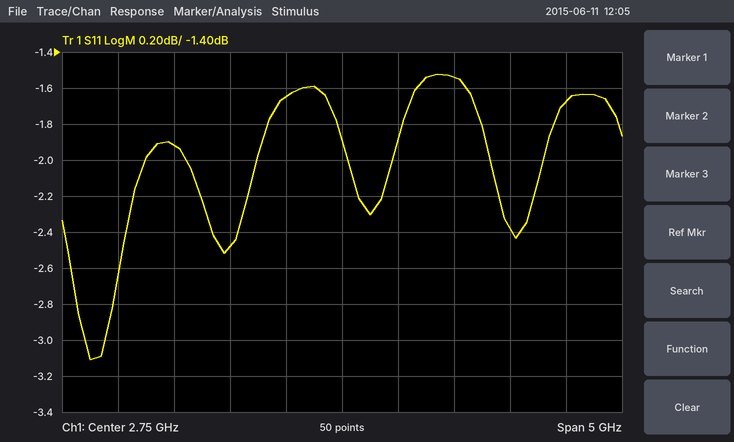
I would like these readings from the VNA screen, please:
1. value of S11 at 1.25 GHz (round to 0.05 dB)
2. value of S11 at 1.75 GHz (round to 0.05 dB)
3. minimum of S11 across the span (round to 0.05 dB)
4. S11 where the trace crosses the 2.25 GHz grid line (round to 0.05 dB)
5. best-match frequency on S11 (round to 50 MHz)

-1.90 dB
-2.50 dB
-3.10 dB
-1.65 dB
500 MHz
